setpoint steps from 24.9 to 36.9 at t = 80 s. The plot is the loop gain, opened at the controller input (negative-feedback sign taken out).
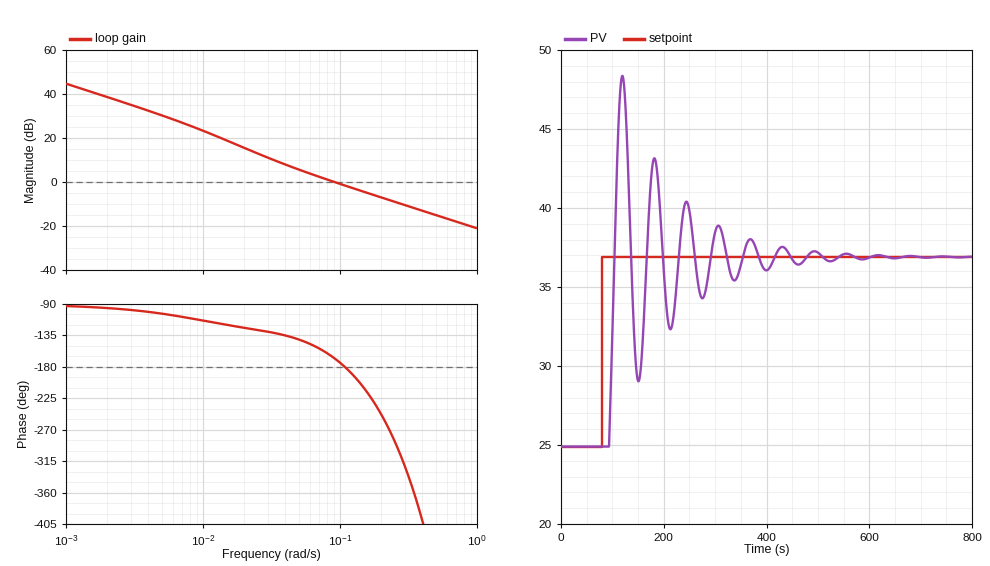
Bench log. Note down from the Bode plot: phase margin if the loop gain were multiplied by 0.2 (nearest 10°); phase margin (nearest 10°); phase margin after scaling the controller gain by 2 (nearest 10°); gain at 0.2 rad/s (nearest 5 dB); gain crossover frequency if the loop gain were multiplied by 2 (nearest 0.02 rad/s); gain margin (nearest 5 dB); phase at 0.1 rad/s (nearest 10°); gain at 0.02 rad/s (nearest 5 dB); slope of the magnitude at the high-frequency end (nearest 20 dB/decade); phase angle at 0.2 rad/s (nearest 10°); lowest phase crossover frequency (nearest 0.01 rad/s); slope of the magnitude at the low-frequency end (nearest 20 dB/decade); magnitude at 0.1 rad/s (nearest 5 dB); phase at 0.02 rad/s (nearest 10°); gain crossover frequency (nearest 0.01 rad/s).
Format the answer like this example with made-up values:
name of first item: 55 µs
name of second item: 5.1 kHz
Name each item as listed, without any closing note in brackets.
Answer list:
phase margin if the loop gain were multiplied by 0.2: 50°
phase margin: 10°
phase margin after scaling the controller gain by 2: -50°
gain at 0.2 rad/s: -5 dB
gain crossover frequency if the loop gain were multiplied by 2: 0.18 rad/s
gain margin: 0 dB
phase at 0.1 rad/s: -170°
gain at 0.02 rad/s: 15 dB
slope of the magnitude at the high-frequency end: -20 dB/decade
phase angle at 0.2 rad/s: -250°
lowest phase crossover frequency: 0.11 rad/s
slope of the magnitude at the low-frequency end: -20 dB/decade
magnitude at 0.1 rad/s: 0 dB
phase at 0.02 rad/s: -120°
gain crossover frequency: 0.09 rad/s
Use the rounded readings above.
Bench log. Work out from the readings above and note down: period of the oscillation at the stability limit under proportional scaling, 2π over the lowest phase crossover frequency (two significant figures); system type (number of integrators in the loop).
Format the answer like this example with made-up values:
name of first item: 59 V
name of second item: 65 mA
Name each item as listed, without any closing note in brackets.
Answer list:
period of the oscillation at the stability limit under proportional scaling, 2π over the lowest phase crossover frequency: 57 s
system type: 1
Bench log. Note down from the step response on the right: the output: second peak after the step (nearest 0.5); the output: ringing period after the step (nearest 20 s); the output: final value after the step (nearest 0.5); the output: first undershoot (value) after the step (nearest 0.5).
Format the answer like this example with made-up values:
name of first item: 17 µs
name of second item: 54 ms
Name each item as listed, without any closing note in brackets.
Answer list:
the output: second peak after the step: 43.0
the output: ringing period after the step: 60 s
the output: final value after the step: 37.0
the output: first undershoot (value) after the step: 29.0
